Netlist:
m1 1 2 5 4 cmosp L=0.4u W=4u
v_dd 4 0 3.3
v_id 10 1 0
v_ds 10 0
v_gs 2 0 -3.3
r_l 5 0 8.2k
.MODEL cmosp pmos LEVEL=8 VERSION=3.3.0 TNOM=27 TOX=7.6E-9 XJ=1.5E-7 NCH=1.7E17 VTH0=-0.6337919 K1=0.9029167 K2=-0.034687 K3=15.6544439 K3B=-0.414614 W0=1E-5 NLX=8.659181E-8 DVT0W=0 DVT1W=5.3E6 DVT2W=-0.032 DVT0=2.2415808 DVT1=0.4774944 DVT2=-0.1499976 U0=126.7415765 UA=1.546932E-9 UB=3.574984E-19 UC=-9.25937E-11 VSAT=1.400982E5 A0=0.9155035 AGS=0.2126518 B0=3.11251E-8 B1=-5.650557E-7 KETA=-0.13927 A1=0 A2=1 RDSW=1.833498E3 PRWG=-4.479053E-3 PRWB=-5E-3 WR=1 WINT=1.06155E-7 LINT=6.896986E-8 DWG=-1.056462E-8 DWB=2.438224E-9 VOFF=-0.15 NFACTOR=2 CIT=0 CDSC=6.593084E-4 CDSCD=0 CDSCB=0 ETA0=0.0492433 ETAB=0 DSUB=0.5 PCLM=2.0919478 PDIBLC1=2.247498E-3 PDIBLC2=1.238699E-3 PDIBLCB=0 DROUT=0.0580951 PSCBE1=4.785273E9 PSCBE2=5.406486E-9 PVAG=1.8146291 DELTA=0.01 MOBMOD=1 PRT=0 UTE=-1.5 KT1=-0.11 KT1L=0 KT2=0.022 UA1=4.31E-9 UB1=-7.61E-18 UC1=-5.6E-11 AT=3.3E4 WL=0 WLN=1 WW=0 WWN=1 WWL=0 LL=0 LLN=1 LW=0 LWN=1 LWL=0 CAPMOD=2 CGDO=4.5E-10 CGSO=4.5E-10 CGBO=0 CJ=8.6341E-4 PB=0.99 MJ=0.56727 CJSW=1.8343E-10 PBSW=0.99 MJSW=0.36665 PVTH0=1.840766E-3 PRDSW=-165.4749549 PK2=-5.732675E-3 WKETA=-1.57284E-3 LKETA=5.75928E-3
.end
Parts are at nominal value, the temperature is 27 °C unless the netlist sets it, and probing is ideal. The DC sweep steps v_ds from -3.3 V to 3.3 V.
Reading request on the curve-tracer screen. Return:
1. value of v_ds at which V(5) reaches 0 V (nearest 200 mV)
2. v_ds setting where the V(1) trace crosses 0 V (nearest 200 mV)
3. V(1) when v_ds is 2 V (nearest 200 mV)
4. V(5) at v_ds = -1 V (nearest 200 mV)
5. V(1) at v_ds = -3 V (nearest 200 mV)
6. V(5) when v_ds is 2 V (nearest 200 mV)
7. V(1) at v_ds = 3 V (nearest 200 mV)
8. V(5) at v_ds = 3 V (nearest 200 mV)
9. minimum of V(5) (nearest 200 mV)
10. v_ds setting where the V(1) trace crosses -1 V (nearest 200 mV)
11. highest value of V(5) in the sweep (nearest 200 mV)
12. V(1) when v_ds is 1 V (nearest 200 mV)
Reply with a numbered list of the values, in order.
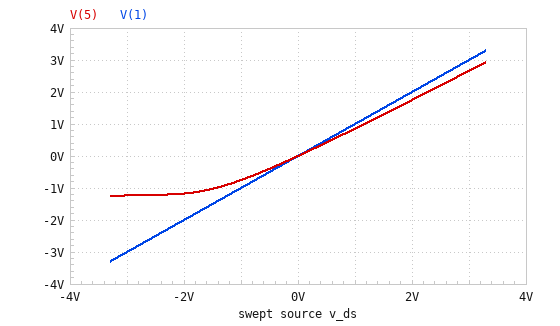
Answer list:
1. 0 V
2. 0 V
3. 2.0 V
4. -800 mV
5. -3.0 V
6. 1.8 V
7. 3.0 V
8. 2.6 V
9. -1.2 V
10. -1.0 V
11. 3.0 V
12. 1.0 V
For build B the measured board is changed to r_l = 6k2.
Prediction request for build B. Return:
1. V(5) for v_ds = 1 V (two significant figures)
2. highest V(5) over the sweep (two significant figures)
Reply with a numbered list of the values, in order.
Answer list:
1. 820 mV
2. 2.8 V
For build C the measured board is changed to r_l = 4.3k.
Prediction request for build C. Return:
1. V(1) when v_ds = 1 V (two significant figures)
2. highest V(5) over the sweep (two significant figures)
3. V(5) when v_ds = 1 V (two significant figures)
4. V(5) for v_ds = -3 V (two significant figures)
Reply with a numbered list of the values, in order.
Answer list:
1. 1.0 V
2. 2.7 V
3. 760 mV
4. -1.0 V
